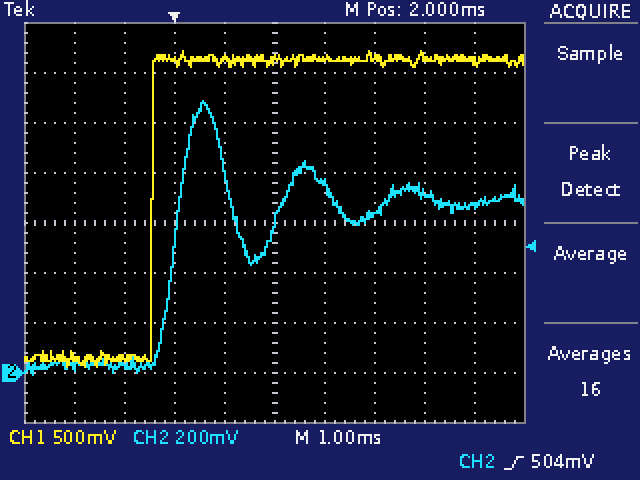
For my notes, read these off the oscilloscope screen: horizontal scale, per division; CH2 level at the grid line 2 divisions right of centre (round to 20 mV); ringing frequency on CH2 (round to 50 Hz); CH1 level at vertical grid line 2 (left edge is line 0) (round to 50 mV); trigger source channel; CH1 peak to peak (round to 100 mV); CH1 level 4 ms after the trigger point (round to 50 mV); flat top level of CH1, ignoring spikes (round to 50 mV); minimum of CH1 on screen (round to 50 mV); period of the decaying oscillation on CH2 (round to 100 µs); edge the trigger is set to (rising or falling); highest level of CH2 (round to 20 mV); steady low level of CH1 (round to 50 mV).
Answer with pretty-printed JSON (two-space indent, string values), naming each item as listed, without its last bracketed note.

{
  "horizontal scale, per division": "1 ms",
  "CH2 level at the grid line 2 divisions right of centre": "640 mV",
  "ringing frequency on CH2": "500 Hz",
  "CH1 level at vertical grid line 2 (left edge is line 0)": "150 mV",
  "trigger source channel": "CH2",
  "CH1 peak to peak": "3.20 V",
  "CH1 level 4 ms after the trigger point": "3.15 V",
  "flat top level of CH1, ignoring spikes": "3.15 V",
  "minimum of CH1 on screen": "50 mV",
  "period of the decaying oscillation on CH2": "2.1 ms",
  "edge the trigger is set to": "rising",
  "highest level of CH2": "1.08 V",
  "steady low level of CH1": "150 mV"
}
